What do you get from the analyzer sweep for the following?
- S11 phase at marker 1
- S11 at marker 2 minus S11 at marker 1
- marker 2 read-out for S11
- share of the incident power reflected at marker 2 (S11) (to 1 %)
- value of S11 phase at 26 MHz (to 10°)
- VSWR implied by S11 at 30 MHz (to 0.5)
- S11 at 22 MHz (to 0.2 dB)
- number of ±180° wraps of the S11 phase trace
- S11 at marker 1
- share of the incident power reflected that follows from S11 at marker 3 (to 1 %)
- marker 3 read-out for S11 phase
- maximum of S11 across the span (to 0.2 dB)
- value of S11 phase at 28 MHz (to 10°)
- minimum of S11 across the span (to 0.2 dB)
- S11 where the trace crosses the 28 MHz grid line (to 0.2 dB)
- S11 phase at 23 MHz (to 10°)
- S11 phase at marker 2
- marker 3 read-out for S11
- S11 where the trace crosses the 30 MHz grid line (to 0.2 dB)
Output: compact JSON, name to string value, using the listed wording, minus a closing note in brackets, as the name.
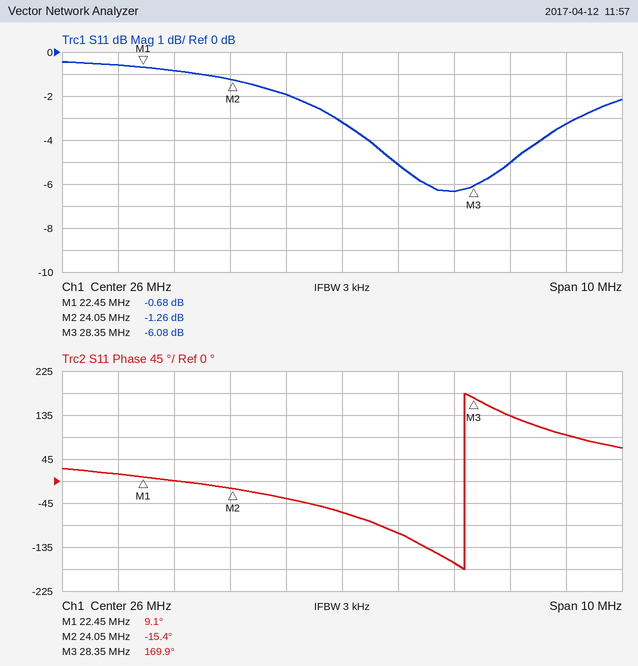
{"S11 phase at marker 1": "9.1°", "S11 at marker 2 minus S11 at marker 1": "-0.58 dB", "marker 2 read-out for S11": "-1.26 dB", "share of the incident power reflected at marker 2 (S11)": "75 %", "value of S11 phase at 26 MHz": "-60°", "VSWR implied by S11 at 30 MHz": "5.5", "S11 at 22 MHz": "-0.6 dB", "number of ±180° wraps of the S11 phase trace": "1", "S11 at marker 1": "-0.68 dB", "share of the incident power reflected that follows from S11 at marker 3": "25 %", "marker 3 read-out for S11 phase": "169.9°", "maximum of S11 across the span": "-0.4 dB", "value of S11 phase at 28 MHz": "-170°", "minimum of S11 across the span": "-6.4 dB", "S11 where the trace crosses the 28 MHz grid line": "-6.4 dB", "S11 phase at 23 MHz": "0°", "S11 phase at marker 2": "-15.4°", "marker 3 read-out for S11": "-6.08 dB", "S11 where the trace crosses the 30 MHz grid line": "-3.2 dB"}
